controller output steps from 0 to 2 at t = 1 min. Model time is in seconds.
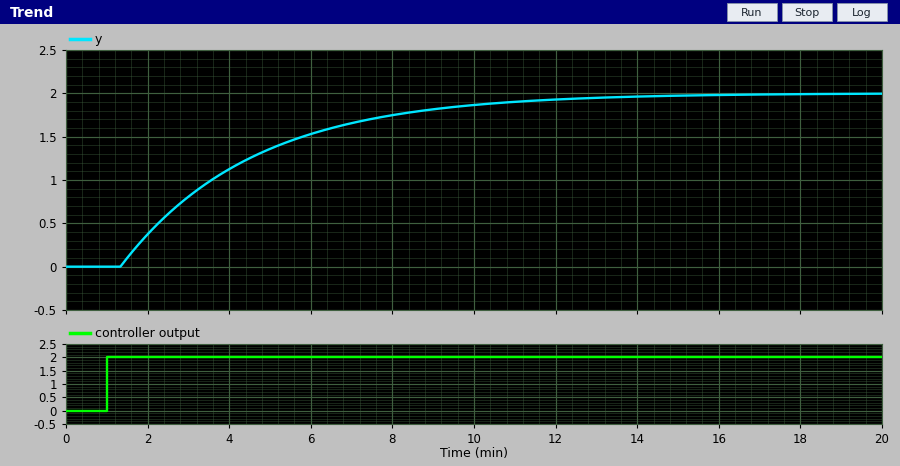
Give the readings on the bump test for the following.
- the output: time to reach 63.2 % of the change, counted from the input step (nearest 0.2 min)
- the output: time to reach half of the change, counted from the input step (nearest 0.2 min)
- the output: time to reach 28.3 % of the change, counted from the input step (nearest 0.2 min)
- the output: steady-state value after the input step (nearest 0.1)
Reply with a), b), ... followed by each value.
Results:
a) 3.6 min
b) 2.6 min
c) 1.4 min
d) 2.0
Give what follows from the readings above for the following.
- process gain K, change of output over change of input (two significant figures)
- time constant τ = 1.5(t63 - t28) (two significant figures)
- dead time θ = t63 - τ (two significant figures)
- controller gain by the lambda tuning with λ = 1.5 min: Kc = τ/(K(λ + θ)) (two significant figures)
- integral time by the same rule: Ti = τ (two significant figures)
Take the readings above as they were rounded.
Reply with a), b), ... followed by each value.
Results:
a) 1.0
b) 3.3 min
c) 0.30 min
d) 1.8
e) 3.3 min
